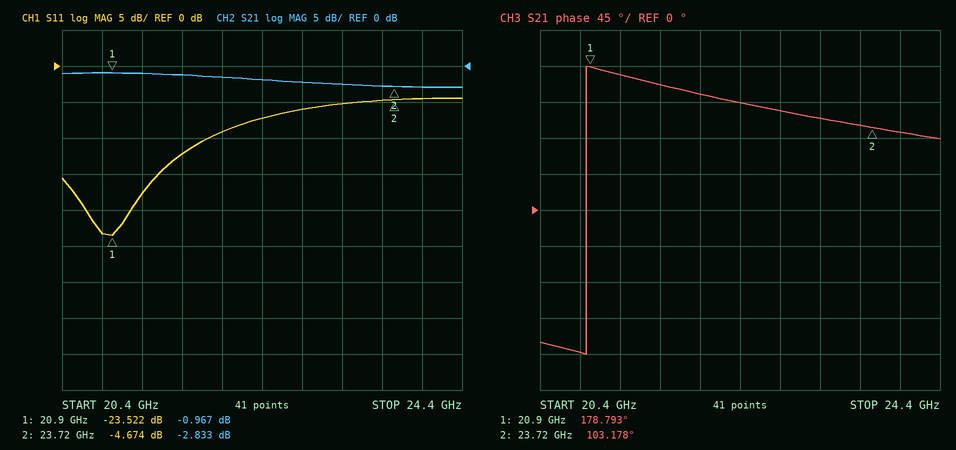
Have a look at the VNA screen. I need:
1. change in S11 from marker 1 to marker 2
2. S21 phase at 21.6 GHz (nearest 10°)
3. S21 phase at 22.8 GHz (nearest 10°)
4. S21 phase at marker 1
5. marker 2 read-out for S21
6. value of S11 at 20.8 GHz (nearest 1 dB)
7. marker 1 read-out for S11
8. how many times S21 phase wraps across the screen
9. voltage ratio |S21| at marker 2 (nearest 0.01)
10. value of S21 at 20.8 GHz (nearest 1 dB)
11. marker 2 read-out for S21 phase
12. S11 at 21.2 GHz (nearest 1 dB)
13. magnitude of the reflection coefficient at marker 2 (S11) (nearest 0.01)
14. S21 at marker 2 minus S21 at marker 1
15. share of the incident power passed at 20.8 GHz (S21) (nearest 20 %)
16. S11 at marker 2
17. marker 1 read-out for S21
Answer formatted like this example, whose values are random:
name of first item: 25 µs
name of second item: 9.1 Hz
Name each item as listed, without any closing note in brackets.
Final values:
change in S11 from marker 1 to marker 2: 18.848 dB
S21 phase at 21.6 GHz: 160°
S21 phase at 22.8 GHz: 120°
S21 phase at marker 1: 178.793°
marker 2 read-out for S21: -2.833 dB
value of S11 at 20.8 GHz: -23 dB
marker 1 read-out for S11: -23.522 dB
how many times S21 phase wraps across the screen: 1
voltage ratio |S21| at marker 2: 0.72
value of S21 at 20.8 GHz: -1 dB
marker 2 read-out for S21 phase: 103.178°
S11 at 21.2 GHz: -18 dB
magnitude of the reflection coefficient at marker 2 (S11): 0.58
S21 at marker 2 minus S21 at marker 1: -1.866 dB
share of the incident power passed at 20.8 GHz (S21): 80 %
S11 at marker 2: -4.674 dB
marker 1 read-out for S21: -0.967 dB
